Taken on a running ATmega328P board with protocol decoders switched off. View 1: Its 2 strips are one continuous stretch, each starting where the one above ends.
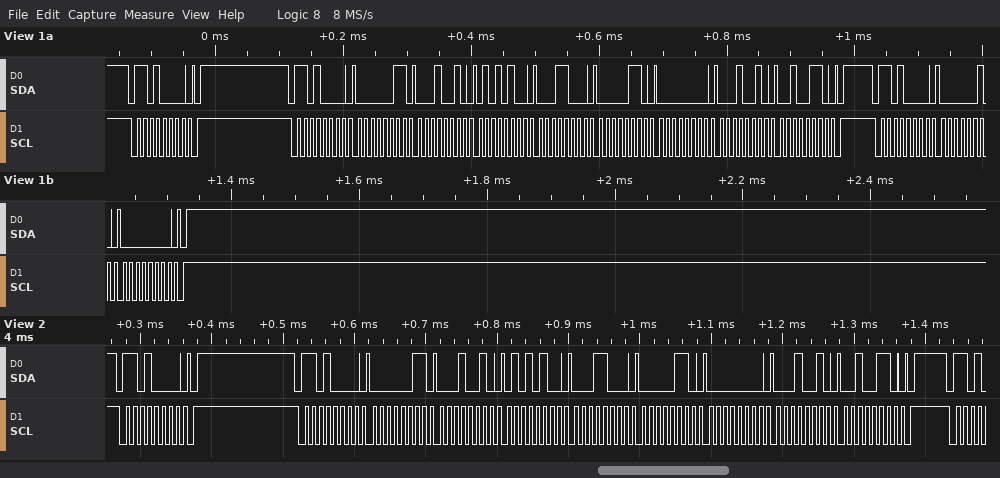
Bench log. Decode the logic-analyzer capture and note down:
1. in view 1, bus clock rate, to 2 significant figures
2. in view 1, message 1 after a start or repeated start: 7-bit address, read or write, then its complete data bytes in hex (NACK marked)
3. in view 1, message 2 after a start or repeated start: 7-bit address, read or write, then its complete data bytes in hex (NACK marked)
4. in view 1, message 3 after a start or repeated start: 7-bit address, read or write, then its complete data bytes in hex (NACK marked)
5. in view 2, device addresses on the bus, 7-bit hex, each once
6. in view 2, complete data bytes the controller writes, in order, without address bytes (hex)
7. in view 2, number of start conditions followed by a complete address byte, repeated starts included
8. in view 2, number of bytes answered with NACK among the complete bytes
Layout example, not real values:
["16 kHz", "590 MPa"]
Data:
["100 kHz", "0x68 write", "0x68 write: 03 12 54 18 06 00 12 26", "0x68 write: 02 00", "0x68", "03 12 54 18 06 00 12 26", "2", "0"]
